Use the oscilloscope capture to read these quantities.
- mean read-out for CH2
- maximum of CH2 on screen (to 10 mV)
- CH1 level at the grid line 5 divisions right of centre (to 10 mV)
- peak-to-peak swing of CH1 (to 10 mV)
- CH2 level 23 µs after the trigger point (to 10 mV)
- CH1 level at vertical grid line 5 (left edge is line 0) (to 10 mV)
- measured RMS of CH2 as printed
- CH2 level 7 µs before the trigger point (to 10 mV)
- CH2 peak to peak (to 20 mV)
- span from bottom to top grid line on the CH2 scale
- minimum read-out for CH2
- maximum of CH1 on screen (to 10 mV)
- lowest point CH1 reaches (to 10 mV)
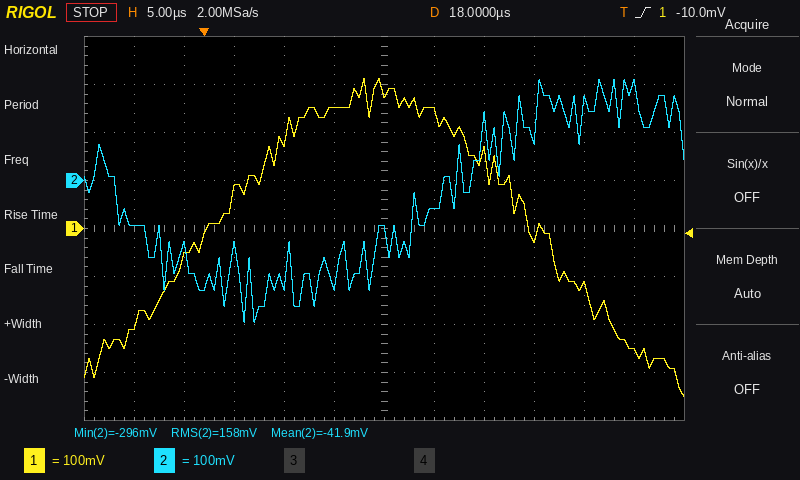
-41.9 mV
210 mV
-260 mV
660 mV
-60 mV
250 mV
158 mV
-90 mV
500 mV
800 mV
-296 mV
310 mV
-350 mV
